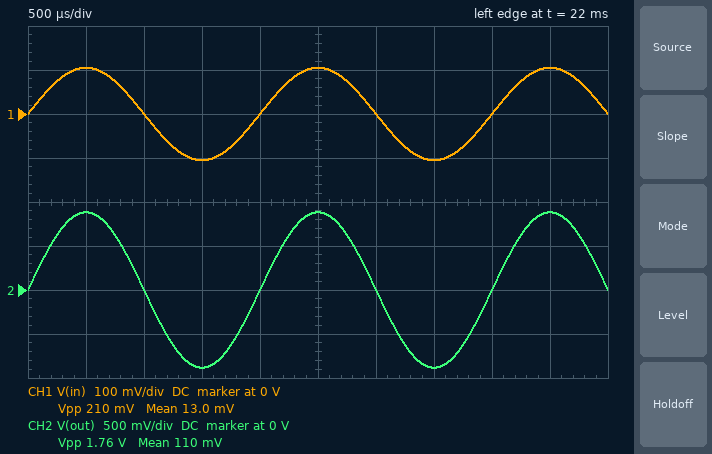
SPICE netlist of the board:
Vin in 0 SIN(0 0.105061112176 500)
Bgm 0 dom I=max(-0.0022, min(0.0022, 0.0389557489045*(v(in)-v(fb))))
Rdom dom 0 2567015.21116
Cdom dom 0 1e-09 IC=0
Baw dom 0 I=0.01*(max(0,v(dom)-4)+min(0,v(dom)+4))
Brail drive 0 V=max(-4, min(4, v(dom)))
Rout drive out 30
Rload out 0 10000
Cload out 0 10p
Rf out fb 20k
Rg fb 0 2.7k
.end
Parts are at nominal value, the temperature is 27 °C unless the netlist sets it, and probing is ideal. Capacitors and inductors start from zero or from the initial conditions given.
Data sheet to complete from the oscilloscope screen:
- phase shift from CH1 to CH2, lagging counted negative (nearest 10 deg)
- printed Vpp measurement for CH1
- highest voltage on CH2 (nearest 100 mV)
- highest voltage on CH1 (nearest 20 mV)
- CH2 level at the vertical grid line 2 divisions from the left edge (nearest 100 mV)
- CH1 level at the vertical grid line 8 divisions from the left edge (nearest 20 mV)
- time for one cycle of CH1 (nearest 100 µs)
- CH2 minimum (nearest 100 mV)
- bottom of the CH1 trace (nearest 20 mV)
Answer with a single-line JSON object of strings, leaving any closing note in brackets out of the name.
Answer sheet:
{"phase shift from CH1 to CH2, lagging counted negative": "0 deg", "printed Vpp measurement for CH1": "210 mV", "highest voltage on CH2": "900 mV", "highest voltage on CH1": "100 mV", "CH2 level at the vertical grid line 2 divisions from the left edge": "0 V", "CH1 level at the vertical grid line 8 divisions from the left edge": "0 V", "time for one cycle of CH1": "2.0 ms", "CH2 minimum": "-900 mV", "bottom of the CH1 trace": "-100 mV"}
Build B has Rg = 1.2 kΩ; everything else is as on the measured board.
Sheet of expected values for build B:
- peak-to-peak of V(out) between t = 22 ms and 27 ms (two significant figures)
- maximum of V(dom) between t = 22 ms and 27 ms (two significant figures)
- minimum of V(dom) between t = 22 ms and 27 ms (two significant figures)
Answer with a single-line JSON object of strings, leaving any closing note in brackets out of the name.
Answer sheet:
{"peak-to-peak of V(out) between t = 22 ms and 27 ms": "3.7 V", "maximum of V(dom) between t = 22 ms and 27 ms": "1.9 V", "minimum of V(dom) between t = 22 ms and 27 ms": "-1.9 V"}
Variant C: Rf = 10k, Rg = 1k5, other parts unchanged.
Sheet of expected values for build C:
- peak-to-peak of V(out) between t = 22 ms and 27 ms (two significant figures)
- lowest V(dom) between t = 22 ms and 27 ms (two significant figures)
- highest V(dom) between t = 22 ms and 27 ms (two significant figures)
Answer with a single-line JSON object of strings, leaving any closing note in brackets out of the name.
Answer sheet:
{"peak-to-peak of V(out) between t = 22 ms and 27 ms": "1.6 V", "lowest V(dom) between t = 22 ms and 27 ms": "-810 mV", "highest V(dom) between t = 22 ms and 27 ms": "810 mV"}
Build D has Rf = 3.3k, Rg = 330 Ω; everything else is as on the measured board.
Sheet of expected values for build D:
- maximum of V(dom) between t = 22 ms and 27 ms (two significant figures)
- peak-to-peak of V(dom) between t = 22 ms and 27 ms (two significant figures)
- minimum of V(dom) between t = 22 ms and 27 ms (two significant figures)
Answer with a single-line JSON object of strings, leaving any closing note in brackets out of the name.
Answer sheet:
{"maximum of V(dom) between t = 22 ms and 27 ms": "1.2 V", "peak-to-peak of V(dom) between t = 22 ms and 27 ms": "2.3 V", "minimum of V(dom) between t = 22 ms and 27 ms": "-1.2 V"}
